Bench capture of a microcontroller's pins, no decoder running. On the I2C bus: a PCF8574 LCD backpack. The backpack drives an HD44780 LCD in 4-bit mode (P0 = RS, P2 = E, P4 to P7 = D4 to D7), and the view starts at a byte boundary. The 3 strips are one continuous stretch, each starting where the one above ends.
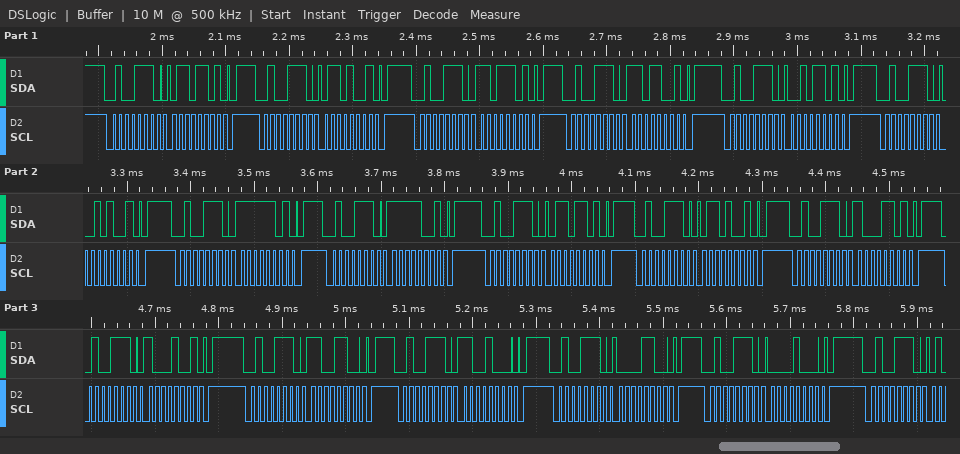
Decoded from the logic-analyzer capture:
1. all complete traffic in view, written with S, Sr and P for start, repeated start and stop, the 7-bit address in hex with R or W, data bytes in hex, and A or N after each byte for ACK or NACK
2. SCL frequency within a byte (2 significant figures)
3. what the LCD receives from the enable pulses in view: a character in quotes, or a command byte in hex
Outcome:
S 27W A 6D A P S 27W A 69 A P S 27W A DD A P S 27W A D9 A P S 27W A 2D A P S 27W A 29 A P S 27W A FD A P S 27W A F9 A P S 27W A 6D A P S 27W A 69 A P S 27W A 8D A P S 27W A 89 A P S 27W A CC A P S 27W A C8 A P S 27W A 0C A P S 27W A 08 A P S 27W A
100 kHz
'm' '/' 'h' 0xC0
